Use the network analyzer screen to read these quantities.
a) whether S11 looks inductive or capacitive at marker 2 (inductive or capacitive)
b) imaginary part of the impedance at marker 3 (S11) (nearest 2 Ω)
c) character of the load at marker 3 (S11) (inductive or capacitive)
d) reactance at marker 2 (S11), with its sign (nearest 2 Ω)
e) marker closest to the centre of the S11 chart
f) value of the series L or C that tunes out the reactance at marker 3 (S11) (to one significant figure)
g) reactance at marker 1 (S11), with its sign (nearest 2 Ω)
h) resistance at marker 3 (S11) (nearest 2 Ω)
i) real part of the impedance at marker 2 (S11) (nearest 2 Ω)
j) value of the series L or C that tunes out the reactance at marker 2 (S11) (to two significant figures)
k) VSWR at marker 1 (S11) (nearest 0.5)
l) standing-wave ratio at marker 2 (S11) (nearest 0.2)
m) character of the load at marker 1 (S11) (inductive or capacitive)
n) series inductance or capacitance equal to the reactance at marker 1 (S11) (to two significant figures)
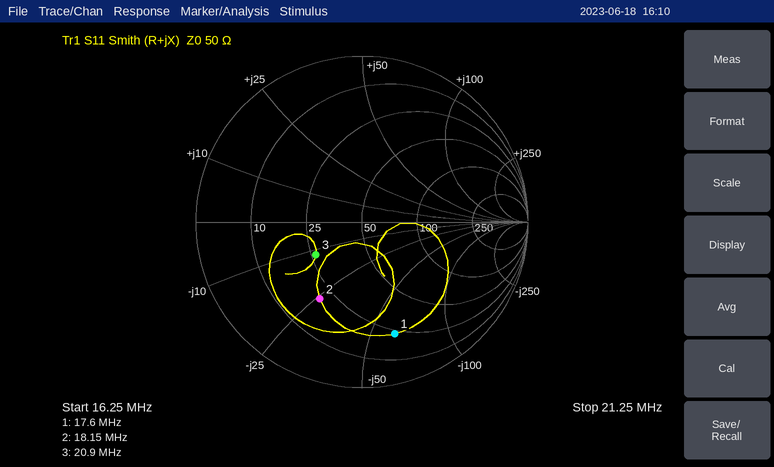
capacitive
-12 Ω
capacitive
-26 Ω
marker 3
90 nH
-62 Ω
26 Ω
20 Ω
230 nH
5.5
3.2
capacitive
150 pF
